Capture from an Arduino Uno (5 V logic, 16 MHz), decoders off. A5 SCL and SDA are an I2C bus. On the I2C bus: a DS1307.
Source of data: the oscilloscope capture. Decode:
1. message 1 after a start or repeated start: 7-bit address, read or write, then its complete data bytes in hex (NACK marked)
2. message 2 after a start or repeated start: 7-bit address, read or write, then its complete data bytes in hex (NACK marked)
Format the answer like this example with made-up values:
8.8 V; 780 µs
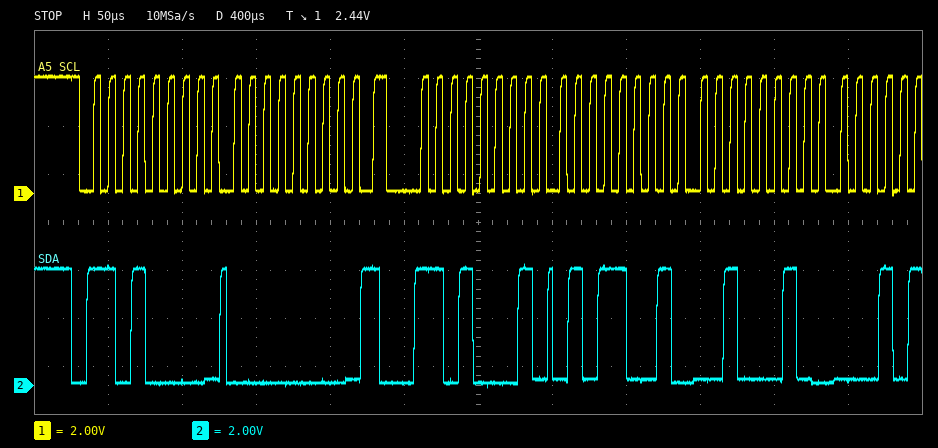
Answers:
0x68 write: 00; 0x68 read: 59 22
